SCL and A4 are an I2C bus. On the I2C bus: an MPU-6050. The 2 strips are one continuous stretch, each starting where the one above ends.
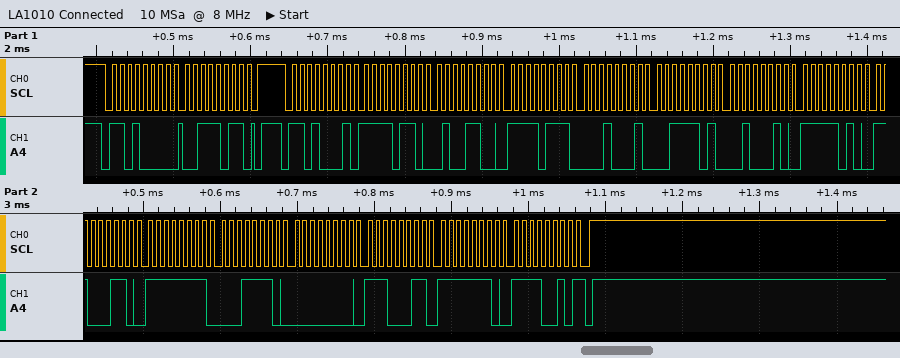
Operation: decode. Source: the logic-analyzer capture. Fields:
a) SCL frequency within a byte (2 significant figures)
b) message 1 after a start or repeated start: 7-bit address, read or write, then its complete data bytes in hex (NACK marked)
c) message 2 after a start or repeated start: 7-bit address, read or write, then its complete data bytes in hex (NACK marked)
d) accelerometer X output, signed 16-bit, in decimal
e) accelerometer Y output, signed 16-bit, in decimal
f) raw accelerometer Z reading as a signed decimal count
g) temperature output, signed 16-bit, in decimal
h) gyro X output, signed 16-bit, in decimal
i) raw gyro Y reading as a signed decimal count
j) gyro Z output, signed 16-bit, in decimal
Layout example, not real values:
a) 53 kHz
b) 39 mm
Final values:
a) 100 kHz
b) 0x68 write: 3B
c) 0x68 read: F6 4C F7 11 3D 22 FA C6 FF 1E 00 E3 FE F2 NACK
d) -2484
e) -2287
f) 15650
g) -1338
h) -226
i) 227
j) -270
